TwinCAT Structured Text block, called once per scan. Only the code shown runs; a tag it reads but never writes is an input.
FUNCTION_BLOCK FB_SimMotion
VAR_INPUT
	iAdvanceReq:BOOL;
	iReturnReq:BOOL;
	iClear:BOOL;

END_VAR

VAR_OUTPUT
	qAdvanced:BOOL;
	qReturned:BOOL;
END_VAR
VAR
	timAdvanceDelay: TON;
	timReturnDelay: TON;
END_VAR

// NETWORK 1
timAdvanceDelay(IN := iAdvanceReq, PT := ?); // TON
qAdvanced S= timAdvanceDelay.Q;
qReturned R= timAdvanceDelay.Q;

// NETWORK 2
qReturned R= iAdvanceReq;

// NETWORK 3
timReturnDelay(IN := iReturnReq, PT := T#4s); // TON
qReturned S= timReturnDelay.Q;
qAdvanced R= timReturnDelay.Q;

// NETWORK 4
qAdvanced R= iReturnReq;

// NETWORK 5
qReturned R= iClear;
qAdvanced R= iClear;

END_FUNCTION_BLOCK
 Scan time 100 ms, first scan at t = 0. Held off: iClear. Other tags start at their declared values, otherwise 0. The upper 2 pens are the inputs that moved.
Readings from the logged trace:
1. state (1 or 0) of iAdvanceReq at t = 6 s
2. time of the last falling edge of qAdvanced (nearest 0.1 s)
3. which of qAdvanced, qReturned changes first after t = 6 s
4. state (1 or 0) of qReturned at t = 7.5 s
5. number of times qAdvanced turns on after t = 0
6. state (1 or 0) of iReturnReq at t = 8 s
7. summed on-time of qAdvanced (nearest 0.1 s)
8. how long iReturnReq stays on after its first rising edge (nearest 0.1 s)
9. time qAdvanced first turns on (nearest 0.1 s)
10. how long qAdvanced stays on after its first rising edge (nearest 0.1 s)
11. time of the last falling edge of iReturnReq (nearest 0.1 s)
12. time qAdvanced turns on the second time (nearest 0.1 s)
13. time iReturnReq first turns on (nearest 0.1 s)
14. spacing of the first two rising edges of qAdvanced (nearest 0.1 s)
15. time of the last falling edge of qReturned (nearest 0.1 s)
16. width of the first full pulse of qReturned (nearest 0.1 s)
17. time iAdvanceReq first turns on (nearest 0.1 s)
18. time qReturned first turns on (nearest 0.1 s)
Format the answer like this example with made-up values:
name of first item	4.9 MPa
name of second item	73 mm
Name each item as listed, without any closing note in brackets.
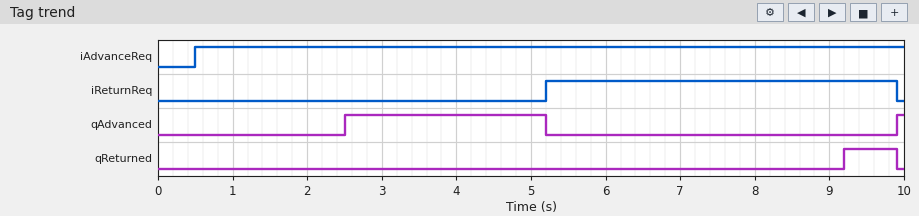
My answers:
state (1 or 0) of iAdvanceReq at t = 6 s	1
time of the last falling edge of qAdvanced	5.2 s
which of qAdvanced, qReturned changes first after t = 6 s	qReturned
state (1 or 0) of qReturned at t = 7.5 s	0
number of times qAdvanced turns on after t = 0	2
state (1 or 0) of iReturnReq at t = 8 s	1
summed on-time of qAdvanced	2.8 s
how long iReturnReq stays on after its first rising edge	4.7 s
time qAdvanced first turns on	2.5 s
how long qAdvanced stays on after its first rising edge	2.7 s
time of the last falling edge of iReturnReq	9.9 s
time qAdvanced turns on the second time	9.9 s
time iReturnReq first turns on	5.2 s
spacing of the first two rising edges of qAdvanced	7.4 s
time of the last falling edge of qReturned	9.9 s
width of the first full pulse of qReturned	0.7 s
time iAdvanceReq first turns on	0.5 s
time qReturned first turns on	9.2 s
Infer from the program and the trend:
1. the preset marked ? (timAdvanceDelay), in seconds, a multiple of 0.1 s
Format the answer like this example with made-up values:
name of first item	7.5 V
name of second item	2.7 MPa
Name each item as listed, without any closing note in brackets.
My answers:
the preset marked ? (timAdvanceDelay), in seconds, a multiple of 0.1 s	2.0 s
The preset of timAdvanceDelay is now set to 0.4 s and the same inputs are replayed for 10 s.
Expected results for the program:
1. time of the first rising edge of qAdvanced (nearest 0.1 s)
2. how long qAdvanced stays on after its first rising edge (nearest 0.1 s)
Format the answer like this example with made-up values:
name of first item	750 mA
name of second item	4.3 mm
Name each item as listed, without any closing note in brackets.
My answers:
time of the first rising edge of qAdvanced	0.9 s
how long qAdvanced stays on after its first rising edge	4.3 s
